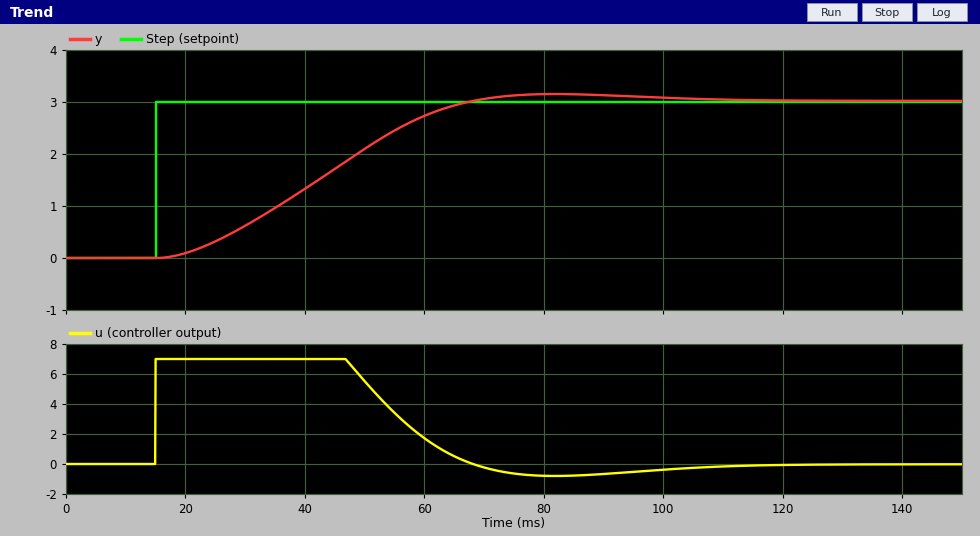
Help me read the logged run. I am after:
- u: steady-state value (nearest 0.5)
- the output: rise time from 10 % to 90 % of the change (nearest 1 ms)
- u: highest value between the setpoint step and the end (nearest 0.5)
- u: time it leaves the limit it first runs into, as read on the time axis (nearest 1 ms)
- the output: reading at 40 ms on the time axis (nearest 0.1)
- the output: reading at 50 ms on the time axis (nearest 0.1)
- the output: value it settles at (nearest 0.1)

0.0
35 ms
7.0
47 ms
1.3
2.1
3.0
